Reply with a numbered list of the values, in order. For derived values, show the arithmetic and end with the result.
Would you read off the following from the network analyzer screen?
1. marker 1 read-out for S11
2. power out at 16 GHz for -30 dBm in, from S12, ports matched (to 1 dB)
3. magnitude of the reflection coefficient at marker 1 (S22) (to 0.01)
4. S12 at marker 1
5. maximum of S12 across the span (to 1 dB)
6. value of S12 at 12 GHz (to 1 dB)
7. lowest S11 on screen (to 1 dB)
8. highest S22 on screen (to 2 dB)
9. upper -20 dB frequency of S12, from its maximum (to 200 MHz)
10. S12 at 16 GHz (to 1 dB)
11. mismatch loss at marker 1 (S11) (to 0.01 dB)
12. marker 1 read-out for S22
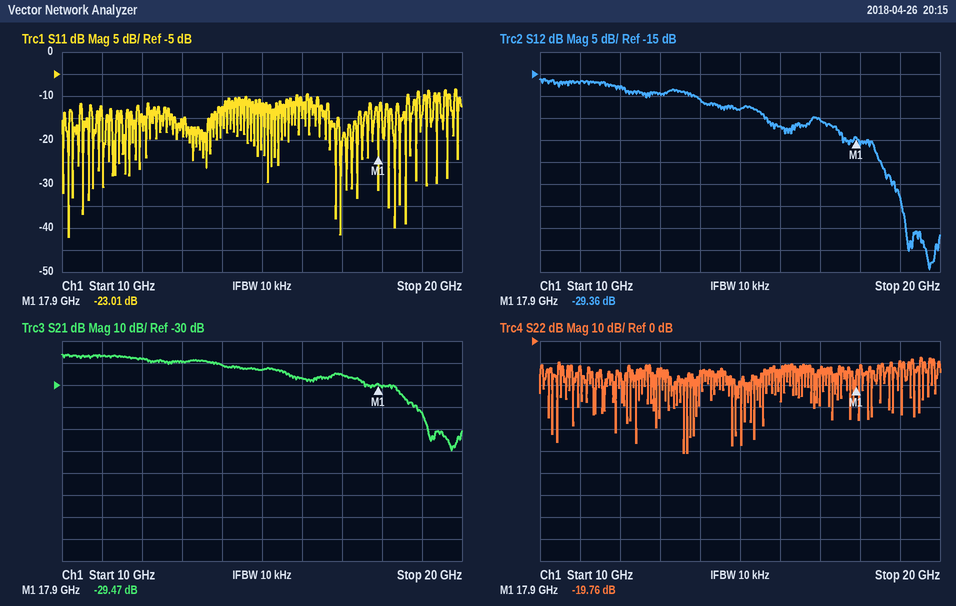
1. -23.01 dB
2. -30 dBm + (-27 dB) = -57 dBm
3. 10^(-19.76/20) ≈ 0.10
4. -29.36 dB
5. -16 dB
6. -18 dB
7. -42 dB
8. -8 dB
9. 18.6 GHz
10. -27 dB
11. −10 log10(1 − 10^(-23.01/10)) ≈ 0.02 dB
12. -19.76 dB
